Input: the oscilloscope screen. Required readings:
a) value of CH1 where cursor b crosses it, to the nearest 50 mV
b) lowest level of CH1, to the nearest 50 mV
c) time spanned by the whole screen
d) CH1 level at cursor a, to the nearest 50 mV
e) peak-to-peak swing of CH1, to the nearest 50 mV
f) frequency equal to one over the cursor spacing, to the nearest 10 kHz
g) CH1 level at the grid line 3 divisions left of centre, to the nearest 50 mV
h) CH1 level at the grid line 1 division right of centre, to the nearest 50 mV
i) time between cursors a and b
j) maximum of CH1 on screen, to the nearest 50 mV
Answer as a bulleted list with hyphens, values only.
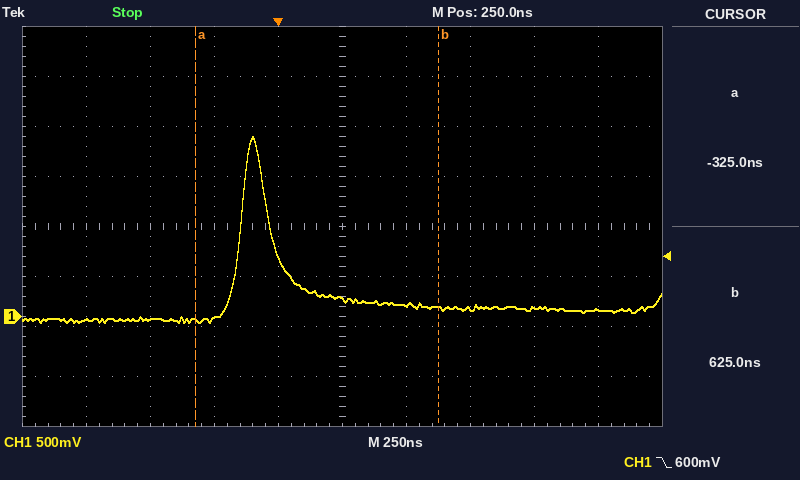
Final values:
- 100 mV
- -50 mV
- 2.5 µs
- -50 mV
- 1.85 V
- 1.05 MHz
- -50 mV
- 100 mV
- 950 ns
- 1.80 V
